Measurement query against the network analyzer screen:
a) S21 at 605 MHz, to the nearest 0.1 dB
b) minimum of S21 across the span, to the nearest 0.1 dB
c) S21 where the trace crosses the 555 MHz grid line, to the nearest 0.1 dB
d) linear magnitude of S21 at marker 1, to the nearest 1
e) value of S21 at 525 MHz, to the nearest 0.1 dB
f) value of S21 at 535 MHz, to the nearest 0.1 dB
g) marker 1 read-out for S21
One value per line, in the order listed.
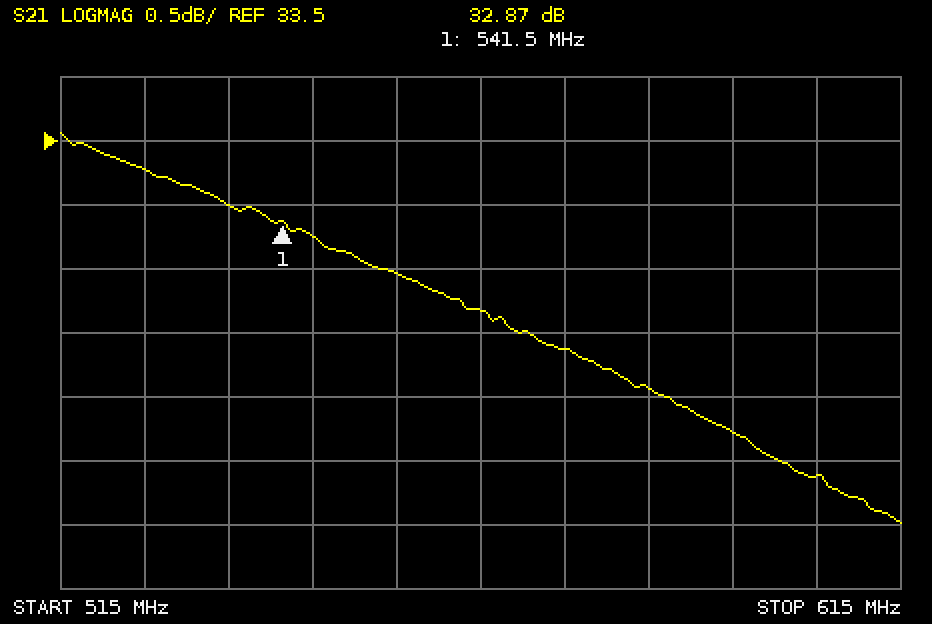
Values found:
30.9 dB
30.5 dB
32.5 dB
44
33.3 dB
33.0 dB
32.87 dB
